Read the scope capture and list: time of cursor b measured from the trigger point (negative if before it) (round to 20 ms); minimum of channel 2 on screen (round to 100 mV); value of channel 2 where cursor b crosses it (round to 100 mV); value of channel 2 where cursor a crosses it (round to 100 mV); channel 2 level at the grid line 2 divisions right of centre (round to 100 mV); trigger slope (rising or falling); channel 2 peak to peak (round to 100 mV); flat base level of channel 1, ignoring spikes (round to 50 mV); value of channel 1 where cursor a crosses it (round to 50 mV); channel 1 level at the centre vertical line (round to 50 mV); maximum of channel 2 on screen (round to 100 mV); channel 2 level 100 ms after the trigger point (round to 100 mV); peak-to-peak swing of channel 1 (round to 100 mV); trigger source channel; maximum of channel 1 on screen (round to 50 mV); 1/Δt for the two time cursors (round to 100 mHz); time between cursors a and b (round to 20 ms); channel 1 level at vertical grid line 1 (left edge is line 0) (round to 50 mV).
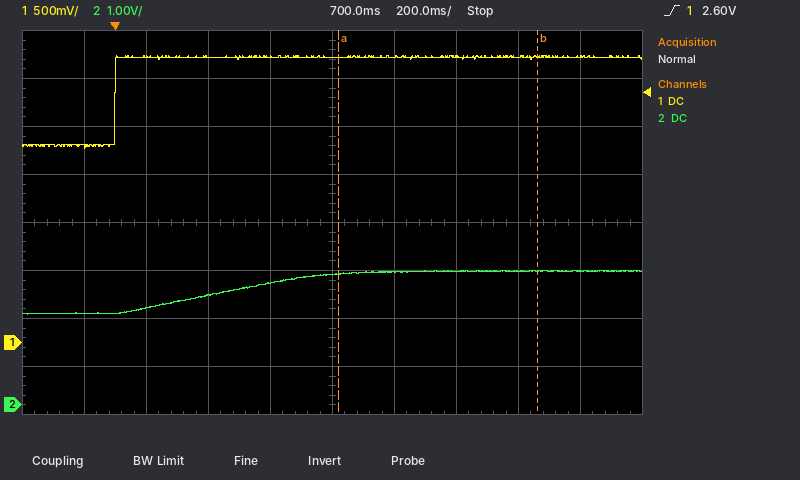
+1.36 s
1.9 V
2.8 V
2.7 V
2.8 V
rising
900 mV
2.05 V
2.95 V
2.95 V
2.8 V
2.0 V
1.00 V
channel 1
3.00 V
1.6 Hz
640 ms
2.05 V
